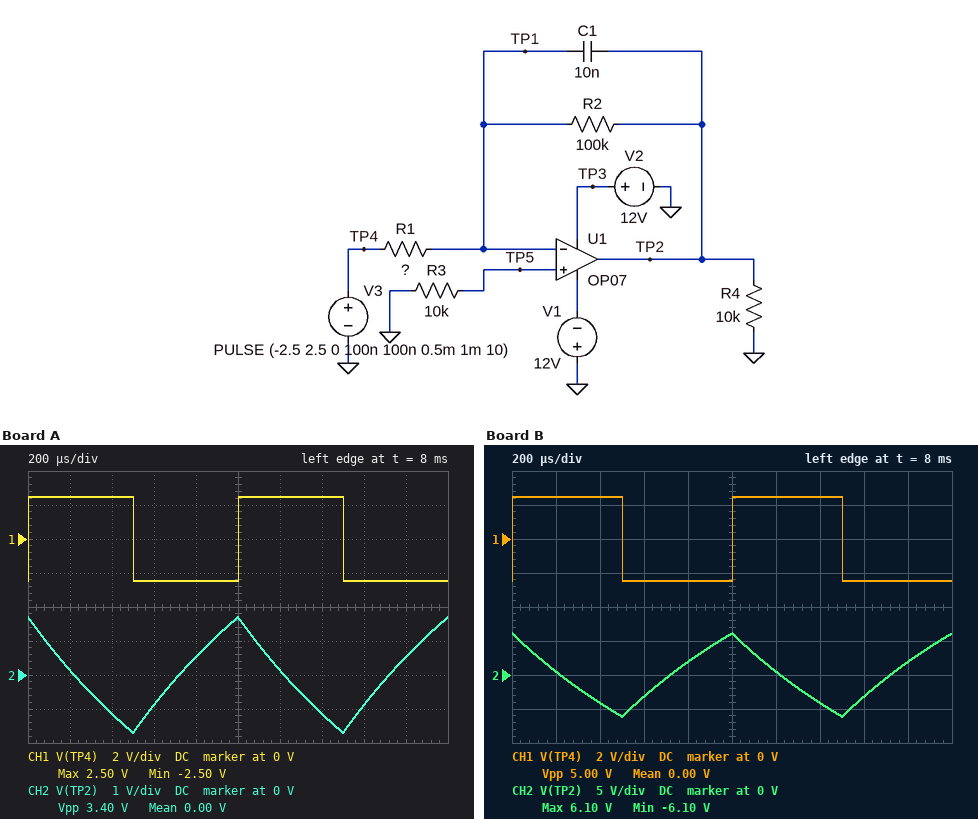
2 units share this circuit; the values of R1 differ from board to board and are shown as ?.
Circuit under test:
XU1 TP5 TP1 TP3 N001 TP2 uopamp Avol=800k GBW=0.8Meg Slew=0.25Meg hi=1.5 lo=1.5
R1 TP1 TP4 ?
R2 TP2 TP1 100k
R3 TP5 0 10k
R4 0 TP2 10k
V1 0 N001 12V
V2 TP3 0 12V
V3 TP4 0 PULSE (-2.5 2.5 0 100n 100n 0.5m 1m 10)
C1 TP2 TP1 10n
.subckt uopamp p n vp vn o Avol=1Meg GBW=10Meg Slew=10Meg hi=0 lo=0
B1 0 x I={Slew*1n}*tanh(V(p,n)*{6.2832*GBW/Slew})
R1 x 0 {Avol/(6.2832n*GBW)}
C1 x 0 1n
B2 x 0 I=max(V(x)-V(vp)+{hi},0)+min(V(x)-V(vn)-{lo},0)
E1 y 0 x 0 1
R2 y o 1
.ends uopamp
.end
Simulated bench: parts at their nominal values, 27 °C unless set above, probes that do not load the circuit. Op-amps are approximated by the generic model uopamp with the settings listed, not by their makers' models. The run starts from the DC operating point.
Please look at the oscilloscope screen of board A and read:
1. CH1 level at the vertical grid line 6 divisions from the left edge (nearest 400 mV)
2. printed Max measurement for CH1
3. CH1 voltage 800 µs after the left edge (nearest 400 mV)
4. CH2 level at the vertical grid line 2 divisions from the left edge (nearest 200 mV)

2.4 V
2.50 V
-2.4 V
-1.2 V
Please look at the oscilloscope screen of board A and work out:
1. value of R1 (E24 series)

36 kΩ
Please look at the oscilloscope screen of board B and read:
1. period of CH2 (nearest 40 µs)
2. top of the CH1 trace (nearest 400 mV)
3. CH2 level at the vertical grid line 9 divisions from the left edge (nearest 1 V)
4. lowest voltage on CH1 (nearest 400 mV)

1.00 ms
2.4 V
2 V
-2.4 V
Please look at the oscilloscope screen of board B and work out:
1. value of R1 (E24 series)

10 kΩ
